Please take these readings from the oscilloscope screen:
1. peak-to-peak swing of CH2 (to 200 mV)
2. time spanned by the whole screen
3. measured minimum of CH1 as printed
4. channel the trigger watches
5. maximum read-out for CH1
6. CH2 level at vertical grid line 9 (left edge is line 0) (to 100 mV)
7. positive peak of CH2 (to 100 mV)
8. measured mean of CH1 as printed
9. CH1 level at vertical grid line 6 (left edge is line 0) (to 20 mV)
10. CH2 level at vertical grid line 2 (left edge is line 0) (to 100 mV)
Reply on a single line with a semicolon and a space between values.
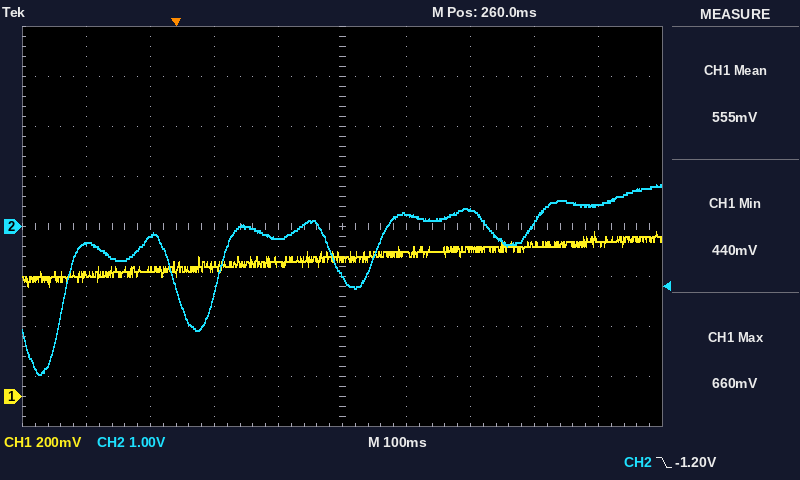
3.8 V; 1 s; 440 mV; CH2; 660 mV; 400 mV; 800 mV; 555 mV; 580 mV; -200 mV
